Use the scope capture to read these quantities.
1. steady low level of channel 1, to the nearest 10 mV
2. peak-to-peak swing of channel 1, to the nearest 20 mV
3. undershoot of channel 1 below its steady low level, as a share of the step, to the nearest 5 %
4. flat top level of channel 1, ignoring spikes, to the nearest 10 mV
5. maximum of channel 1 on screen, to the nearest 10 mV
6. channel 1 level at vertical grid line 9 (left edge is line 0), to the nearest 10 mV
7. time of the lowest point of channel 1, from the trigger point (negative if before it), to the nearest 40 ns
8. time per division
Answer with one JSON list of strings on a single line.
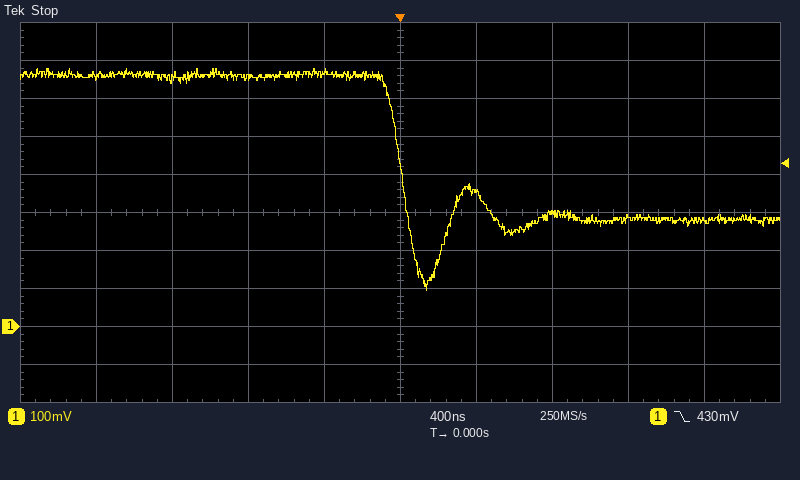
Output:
["280 mV", "580 mV", "50 %", "660 mV", "680 mV", "280 mV", "+120 ns", "400 ns"]
